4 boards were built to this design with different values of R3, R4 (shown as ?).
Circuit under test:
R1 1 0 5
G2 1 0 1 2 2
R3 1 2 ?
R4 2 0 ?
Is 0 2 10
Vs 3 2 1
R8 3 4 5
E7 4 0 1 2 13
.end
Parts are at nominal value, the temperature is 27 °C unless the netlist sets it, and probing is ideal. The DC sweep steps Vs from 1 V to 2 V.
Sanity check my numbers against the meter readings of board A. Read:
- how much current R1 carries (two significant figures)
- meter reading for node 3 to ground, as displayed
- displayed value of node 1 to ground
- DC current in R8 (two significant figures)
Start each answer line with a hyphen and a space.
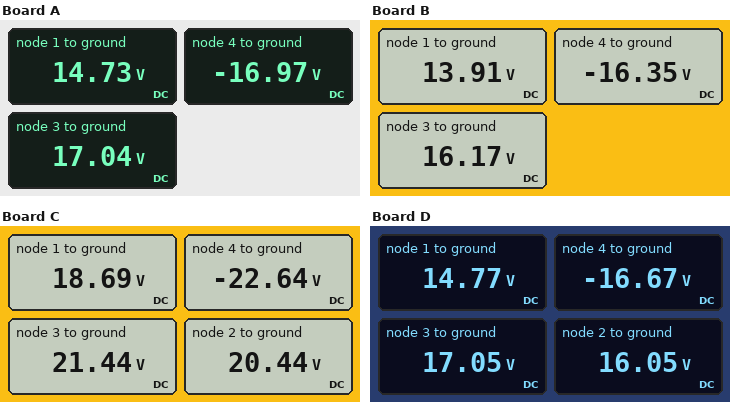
- 2.9 A
- 17.04 V
- 14.73 V
- 6.8 A
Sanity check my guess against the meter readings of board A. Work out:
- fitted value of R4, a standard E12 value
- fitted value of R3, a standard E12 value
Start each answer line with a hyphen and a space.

- 5.6 Ω
- 3.9 Ω
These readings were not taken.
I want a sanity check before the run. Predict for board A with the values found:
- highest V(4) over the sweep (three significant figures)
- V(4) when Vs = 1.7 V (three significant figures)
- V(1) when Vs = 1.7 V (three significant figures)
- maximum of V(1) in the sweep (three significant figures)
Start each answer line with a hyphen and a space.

- -16.6 V
- -16.7 V
- 14.5 V
- 14.7 V
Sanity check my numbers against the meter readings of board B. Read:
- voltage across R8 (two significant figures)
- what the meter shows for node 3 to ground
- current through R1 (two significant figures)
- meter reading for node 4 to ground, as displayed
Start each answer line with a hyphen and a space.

- 33 V
- 16.17 V
- 2.8 A
- -16.35 V
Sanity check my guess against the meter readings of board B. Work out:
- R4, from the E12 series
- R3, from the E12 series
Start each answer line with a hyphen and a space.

- 4.7 Ω
- 4.7 Ω
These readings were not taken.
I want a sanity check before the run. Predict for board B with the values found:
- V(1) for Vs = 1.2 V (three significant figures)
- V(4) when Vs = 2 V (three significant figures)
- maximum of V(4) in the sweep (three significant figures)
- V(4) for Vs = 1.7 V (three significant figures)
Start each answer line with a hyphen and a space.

- 13.9 V
- -16.0 V
- -16.0 V
- -16.1 V
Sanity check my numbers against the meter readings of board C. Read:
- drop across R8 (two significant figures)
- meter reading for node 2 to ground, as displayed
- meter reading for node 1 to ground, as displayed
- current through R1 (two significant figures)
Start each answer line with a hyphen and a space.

- 44 V
- 20.44 V
- 18.69 V
- 3.7 A
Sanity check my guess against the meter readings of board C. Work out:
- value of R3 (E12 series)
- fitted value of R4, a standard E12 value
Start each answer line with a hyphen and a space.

- 6.8 Ω
- 22 Ω
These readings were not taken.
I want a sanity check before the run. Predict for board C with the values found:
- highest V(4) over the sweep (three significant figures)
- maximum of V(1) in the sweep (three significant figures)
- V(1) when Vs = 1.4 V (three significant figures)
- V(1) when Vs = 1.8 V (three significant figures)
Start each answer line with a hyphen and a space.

- -22.2 V
- 18.7 V
- 18.5 V
- 18.4 V
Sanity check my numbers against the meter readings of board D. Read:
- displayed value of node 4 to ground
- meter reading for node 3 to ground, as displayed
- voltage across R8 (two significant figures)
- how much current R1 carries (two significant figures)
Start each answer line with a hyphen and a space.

- -16.67 V
- 17.05 V
- 34 V
- 3.0 A
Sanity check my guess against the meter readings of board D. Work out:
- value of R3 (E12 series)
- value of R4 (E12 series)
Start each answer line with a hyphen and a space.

- 3.3 Ω
- 5.6 Ω
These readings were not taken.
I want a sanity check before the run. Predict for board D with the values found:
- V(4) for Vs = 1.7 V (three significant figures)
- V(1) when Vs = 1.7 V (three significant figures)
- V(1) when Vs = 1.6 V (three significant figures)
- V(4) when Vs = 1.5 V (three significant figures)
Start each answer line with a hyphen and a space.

- -16.4 V
- 14.6 V
- 14.6 V
- -16.5 V
